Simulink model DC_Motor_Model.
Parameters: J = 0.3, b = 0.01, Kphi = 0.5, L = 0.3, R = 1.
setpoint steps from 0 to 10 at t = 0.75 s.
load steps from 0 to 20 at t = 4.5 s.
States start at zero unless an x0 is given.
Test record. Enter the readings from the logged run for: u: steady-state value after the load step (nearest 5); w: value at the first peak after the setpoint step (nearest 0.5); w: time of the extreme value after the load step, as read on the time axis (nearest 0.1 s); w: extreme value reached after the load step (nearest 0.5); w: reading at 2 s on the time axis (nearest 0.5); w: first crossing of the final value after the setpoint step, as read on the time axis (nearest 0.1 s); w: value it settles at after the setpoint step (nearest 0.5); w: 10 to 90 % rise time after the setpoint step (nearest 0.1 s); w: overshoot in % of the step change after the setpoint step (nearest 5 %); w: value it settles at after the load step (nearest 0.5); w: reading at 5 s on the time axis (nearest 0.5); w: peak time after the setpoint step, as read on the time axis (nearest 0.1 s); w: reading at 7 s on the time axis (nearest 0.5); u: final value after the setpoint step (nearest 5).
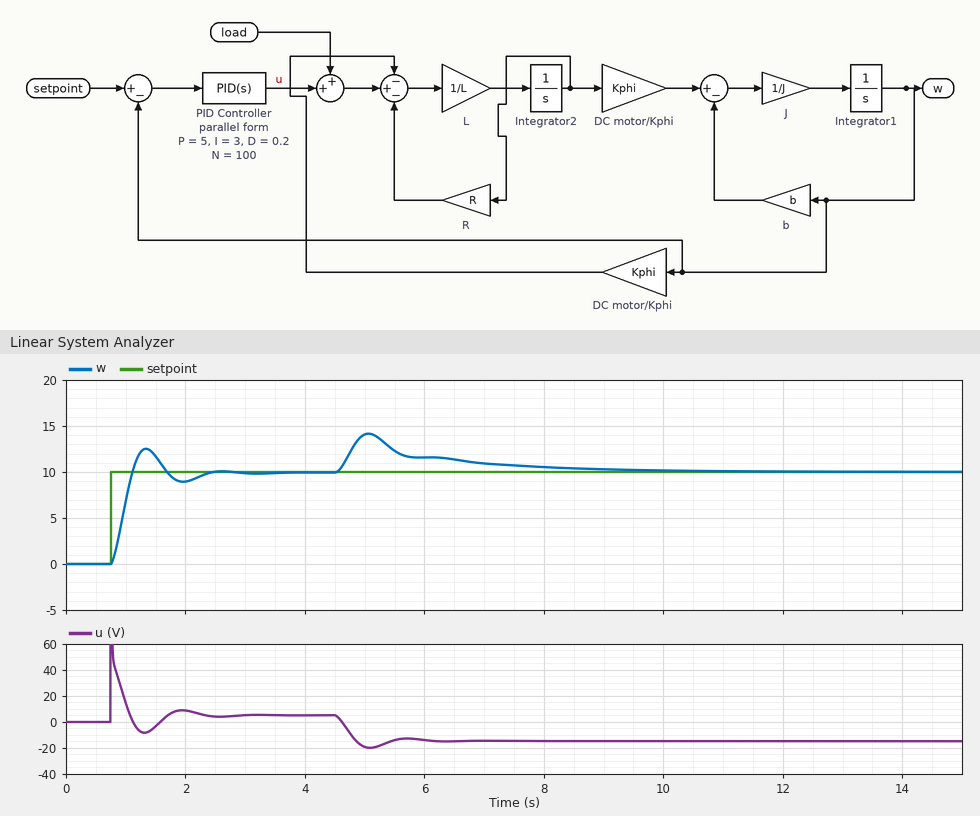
-15
12.5
5.1 s
14.0
9.0
1.1 s
10.0
0.3 s
25 %
10.0
14.0
1.3 s
11.0
5
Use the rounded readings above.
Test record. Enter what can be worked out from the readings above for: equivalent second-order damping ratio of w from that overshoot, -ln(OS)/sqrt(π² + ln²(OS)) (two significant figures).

0.40
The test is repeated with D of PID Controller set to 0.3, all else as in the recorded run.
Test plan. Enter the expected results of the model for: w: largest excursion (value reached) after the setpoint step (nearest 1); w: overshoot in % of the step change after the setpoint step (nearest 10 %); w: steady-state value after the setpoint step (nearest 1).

12
20 %
10
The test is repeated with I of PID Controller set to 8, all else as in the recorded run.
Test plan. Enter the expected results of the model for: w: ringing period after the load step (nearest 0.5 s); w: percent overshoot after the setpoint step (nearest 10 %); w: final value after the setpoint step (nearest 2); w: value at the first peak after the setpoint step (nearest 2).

1.5 s
40 %
10
14
